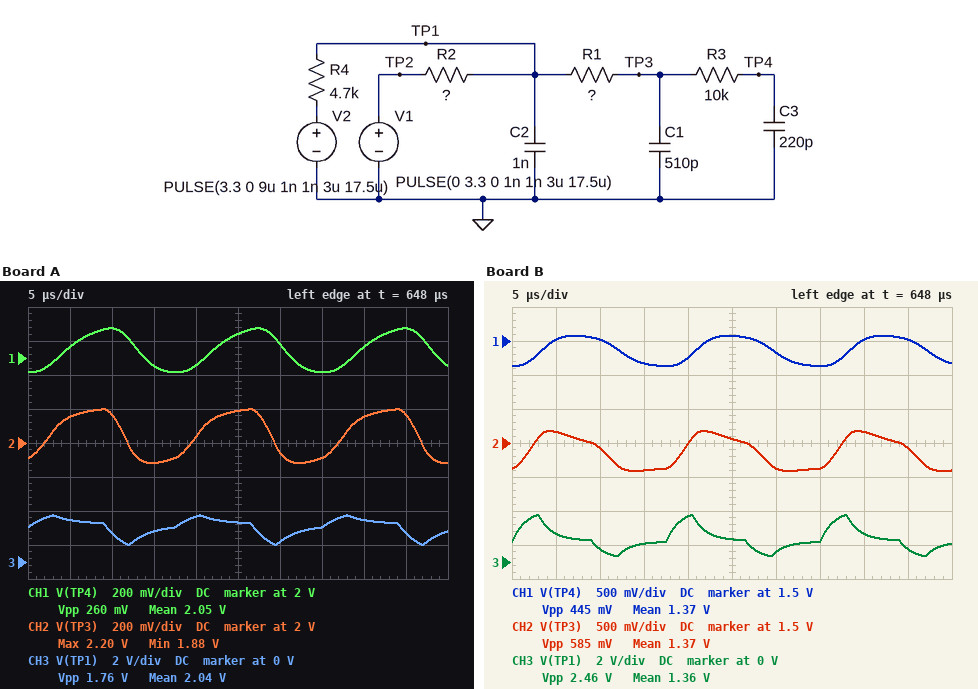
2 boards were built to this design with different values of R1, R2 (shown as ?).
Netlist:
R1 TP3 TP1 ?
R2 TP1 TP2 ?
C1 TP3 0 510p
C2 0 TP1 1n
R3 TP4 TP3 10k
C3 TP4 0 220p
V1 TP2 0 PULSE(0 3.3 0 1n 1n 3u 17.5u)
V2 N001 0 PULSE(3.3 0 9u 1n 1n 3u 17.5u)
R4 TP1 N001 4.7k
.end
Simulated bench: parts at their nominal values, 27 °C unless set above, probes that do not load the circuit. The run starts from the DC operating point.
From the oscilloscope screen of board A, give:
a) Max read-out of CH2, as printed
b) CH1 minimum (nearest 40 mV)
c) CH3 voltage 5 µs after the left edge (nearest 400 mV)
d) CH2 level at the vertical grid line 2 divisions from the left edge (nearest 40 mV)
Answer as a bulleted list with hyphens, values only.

- 2.20 V
- 1.92 V
- 2.4 V
- 2.16 V
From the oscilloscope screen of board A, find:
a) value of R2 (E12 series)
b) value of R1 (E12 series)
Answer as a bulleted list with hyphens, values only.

- 10 kΩ
- 15 kΩ
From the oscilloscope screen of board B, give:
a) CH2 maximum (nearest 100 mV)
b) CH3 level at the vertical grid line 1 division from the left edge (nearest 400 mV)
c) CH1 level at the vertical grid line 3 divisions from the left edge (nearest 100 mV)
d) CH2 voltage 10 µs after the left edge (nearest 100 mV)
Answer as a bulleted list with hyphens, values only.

- 1.7 V
- 1.6 V
- 1.2 V
- 1.4 V
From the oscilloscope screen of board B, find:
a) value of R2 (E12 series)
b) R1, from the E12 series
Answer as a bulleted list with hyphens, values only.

- 2.7 kΩ
- 10 kΩ
